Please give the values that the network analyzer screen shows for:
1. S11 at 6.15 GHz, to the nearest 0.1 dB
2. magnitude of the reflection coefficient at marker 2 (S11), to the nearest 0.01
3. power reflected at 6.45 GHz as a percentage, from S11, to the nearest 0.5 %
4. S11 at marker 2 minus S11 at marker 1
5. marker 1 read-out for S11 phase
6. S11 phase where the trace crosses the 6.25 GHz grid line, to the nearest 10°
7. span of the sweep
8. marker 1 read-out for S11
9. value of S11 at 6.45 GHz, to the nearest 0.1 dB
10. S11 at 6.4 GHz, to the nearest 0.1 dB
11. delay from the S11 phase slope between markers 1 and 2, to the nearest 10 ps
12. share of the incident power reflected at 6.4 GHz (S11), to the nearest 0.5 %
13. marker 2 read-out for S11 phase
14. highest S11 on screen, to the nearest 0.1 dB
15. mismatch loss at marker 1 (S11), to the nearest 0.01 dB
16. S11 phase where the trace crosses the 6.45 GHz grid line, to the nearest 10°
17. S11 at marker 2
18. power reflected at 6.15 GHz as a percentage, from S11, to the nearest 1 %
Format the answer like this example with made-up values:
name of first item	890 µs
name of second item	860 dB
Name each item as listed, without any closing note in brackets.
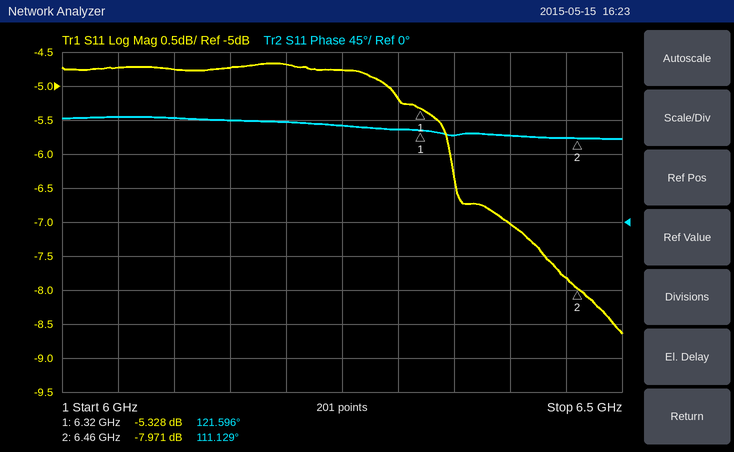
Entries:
S11 at 6.15 GHz, to the nearest 0.1 dB	-4.7 dB
magnitude of the reflection coefficient at marker 2 (S11), to the nearest 0.01	0.40
power reflected at 6.45 GHz as a percentage, from S11, to the nearest 0.5 %	16.5 %
S11 at marker 2 minus S11 at marker 1	-2.643 dB
marker 1 read-out for S11 phase	121.596°
S11 phase where the trace crosses the 6.25 GHz grid line, to the nearest 10°	130°
span of the sweep	500 MHz
marker 1 read-out for S11	-5.328 dB
value of S11 at 6.45 GHz, to the nearest 0.1 dB	-7.8 dB
S11 at 6.4 GHz, to the nearest 0.1 dB	-7.0 dB
delay from the S11 phase slope between markers 1 and 2, to the nearest 10 ps	210 ps
share of the incident power reflected at 6.4 GHz (S11), to the nearest 0.5 %	20.0 %
marker 2 read-out for S11 phase	111.129°
highest S11 on screen, to the nearest 0.1 dB	-4.7 dB
mismatch loss at marker 1 (S11), to the nearest 0.01 dB	1.51 dB
S11 phase where the trace crosses the 6.45 GHz grid line, to the nearest 10°	110°
S11 at marker 2	-7.971 dB
power reflected at 6.15 GHz as a percentage, from S11, to the nearest 1 %	34 %
